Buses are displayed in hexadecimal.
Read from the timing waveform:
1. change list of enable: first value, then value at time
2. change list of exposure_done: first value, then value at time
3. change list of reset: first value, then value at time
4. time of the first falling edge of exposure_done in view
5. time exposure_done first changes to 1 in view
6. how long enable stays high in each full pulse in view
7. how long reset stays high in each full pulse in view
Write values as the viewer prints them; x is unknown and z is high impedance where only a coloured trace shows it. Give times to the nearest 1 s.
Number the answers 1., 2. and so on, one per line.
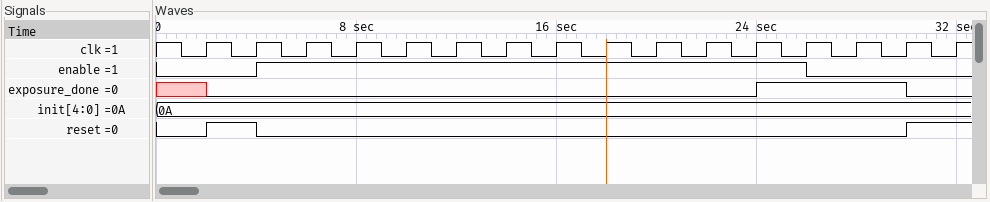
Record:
1. 0, 1 at 4 s, 0 at 26 s
2. x, 0 at 2 s, 1 at 24 s, 0 at 30 s
3. 0, 1 at 2 s, 0 at 4 s, 1 at 30 s
4. 30 s
5. 24 s
6. 22 s
7. 2 s
